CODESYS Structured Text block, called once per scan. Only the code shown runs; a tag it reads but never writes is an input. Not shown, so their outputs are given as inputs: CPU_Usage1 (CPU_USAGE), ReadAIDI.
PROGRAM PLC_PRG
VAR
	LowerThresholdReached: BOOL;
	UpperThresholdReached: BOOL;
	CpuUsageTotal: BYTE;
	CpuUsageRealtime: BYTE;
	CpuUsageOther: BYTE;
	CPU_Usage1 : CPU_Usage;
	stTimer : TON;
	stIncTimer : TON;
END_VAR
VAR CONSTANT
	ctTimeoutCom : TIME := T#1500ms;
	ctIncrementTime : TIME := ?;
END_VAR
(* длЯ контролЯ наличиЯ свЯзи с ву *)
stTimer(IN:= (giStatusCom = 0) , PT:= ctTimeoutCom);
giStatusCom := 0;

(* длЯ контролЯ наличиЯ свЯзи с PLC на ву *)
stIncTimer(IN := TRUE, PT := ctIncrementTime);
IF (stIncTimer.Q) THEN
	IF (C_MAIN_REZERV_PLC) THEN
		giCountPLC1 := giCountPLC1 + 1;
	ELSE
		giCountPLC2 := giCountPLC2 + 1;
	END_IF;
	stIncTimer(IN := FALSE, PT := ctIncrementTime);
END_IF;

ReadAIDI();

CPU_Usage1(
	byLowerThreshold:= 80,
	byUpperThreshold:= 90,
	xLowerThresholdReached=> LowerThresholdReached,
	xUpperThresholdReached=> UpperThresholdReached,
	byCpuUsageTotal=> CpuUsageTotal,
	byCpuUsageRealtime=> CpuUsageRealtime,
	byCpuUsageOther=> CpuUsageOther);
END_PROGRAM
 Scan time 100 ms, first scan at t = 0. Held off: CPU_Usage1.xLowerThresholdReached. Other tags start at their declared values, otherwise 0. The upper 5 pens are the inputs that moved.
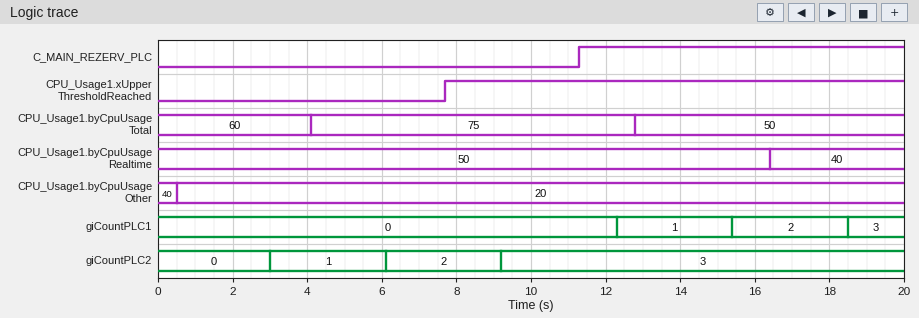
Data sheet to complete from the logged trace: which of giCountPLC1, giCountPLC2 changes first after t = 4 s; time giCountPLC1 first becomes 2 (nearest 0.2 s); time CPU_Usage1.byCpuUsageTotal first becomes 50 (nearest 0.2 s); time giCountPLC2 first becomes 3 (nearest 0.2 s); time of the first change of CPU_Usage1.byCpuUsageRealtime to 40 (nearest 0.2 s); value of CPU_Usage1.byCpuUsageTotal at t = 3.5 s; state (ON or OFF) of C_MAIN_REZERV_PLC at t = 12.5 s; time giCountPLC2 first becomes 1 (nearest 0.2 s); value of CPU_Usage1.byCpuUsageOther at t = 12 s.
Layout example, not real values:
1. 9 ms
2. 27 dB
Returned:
1. giCountPLC2
2. 15.4 s
3. 12.8 s
4. 9.2 s
5. 16.4 s
6. 60
7. ON
8. 3.0 s
9. 20
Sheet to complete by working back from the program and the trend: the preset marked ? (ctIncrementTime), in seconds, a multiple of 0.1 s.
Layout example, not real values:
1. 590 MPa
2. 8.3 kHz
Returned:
1. 3.0 s
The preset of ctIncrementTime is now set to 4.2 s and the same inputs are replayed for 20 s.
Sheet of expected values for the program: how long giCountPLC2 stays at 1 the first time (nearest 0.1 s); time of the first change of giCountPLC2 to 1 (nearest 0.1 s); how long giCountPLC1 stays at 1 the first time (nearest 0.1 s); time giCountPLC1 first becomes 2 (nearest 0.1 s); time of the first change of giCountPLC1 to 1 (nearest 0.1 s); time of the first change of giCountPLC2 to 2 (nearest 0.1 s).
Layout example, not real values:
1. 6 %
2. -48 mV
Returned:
1. 4.3 s
2. 4.2 s
3. 4.3 s
4. 17.1 s
5. 12.8 s
6. 8.5 s
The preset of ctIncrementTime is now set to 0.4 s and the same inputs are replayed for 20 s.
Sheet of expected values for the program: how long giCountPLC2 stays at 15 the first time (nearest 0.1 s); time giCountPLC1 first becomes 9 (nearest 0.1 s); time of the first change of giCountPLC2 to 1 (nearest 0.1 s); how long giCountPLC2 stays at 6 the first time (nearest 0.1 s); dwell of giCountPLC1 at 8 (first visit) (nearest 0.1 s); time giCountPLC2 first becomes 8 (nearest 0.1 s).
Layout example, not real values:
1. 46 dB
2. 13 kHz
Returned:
1. 0.5 s
2. 15.4 s
3. 0.4 s
4. 0.5 s
5. 0.5 s
6. 3.9 s
